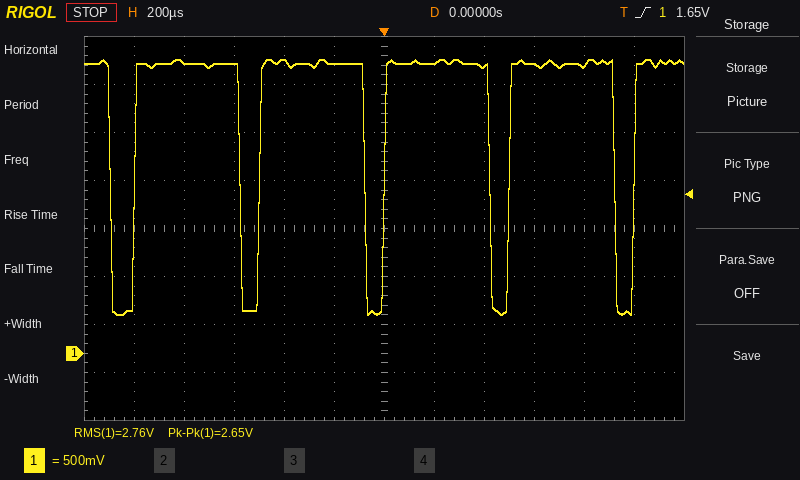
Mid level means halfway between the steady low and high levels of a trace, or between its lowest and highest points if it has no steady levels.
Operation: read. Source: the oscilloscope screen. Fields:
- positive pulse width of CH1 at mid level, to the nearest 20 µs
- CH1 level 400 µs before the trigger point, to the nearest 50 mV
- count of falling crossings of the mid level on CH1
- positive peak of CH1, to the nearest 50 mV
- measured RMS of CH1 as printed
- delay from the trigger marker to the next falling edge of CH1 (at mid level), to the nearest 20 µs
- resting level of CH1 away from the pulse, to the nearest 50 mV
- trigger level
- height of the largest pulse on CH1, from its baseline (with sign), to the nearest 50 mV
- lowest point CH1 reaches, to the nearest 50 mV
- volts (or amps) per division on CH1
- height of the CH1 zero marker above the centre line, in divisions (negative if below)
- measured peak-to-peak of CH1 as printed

420 µs
3.05 V
5
3.05 V
2.76 V
420 µs
3.00 V
1.65 V
-2.60 V
400 mV
500 mV
-2.6 div
2.65 V
